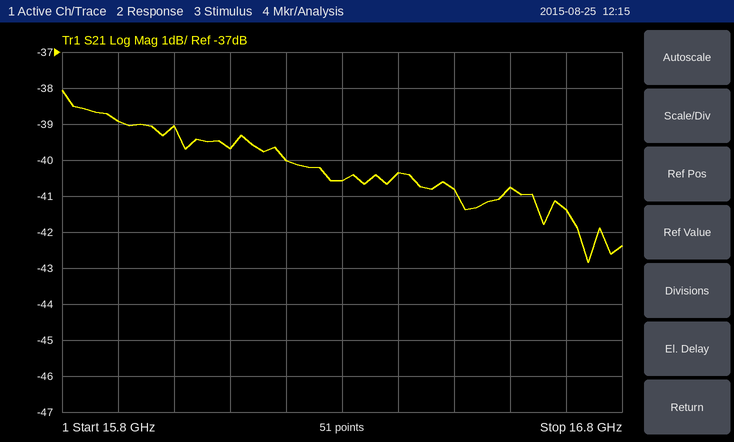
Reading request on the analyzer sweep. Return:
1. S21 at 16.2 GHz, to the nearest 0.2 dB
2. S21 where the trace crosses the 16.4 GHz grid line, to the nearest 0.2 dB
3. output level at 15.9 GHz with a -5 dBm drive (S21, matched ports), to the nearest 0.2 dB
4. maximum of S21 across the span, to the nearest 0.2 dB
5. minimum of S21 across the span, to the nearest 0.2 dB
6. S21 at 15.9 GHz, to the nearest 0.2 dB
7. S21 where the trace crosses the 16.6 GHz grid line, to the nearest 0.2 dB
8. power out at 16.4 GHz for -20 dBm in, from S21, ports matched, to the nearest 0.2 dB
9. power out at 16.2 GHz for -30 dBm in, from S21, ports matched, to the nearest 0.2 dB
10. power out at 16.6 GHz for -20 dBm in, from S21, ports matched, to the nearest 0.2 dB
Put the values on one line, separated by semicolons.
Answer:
-40.0 dB; -40.4 dB; -44.0 dBm; -38.0 dB; -42.8 dB; -39.0 dB; -40.8 dB; -60.4 dBm; -70.0 dBm; -60.8 dBm
